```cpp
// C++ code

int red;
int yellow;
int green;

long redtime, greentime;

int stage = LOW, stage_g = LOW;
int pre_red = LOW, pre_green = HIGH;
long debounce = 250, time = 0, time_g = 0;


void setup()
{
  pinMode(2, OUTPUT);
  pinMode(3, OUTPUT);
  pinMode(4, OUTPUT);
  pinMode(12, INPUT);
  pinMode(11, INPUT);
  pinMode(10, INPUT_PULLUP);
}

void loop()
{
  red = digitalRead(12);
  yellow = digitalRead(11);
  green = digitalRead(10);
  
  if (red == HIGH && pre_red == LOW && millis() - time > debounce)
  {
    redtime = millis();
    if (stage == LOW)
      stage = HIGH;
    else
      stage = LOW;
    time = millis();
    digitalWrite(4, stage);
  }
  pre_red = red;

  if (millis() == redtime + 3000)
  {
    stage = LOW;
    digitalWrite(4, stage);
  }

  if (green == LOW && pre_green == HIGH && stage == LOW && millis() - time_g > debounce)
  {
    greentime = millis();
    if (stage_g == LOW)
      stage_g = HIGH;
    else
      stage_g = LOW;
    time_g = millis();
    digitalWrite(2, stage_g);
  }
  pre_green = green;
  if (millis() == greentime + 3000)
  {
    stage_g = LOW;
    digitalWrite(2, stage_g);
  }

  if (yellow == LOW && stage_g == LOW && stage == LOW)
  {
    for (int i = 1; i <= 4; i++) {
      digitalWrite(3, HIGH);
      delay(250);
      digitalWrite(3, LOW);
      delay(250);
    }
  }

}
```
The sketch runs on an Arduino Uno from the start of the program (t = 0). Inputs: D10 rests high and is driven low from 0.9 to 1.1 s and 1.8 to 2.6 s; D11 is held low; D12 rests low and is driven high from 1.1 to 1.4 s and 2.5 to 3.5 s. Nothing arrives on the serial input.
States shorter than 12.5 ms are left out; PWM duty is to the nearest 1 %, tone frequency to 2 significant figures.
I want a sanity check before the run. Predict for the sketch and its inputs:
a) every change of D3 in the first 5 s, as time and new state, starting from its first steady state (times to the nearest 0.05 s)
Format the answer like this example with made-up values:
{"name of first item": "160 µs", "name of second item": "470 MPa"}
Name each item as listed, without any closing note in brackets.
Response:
{"every change of D3 in the first 5 s, as time and new state, starting from its first steady state": "0 s high; 0.25 s low; 0.5 s high; 0.75 s low; 1 s high; 1.25 s low; 1.5 s high; 1.75 s low"}
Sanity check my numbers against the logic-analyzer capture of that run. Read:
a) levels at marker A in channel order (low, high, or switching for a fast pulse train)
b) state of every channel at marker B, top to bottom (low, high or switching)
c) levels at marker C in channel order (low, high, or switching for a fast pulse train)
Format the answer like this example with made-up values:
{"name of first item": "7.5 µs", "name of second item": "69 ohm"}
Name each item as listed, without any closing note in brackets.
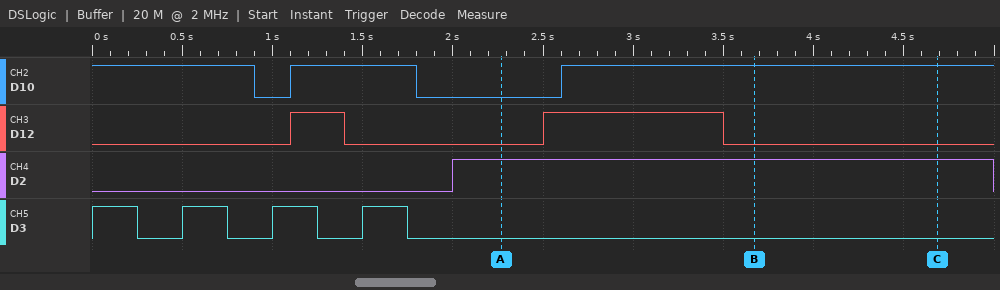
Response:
{"levels at marker A in channel order": "D10 low, D12 low, D2 high, D3 low", "state of every channel at marker B, top to bottom": "D10 high, D12 low, D2 high, D3 low", "levels at marker C in channel order": "D10 high, D12 low, D2 high, D3 low"}
